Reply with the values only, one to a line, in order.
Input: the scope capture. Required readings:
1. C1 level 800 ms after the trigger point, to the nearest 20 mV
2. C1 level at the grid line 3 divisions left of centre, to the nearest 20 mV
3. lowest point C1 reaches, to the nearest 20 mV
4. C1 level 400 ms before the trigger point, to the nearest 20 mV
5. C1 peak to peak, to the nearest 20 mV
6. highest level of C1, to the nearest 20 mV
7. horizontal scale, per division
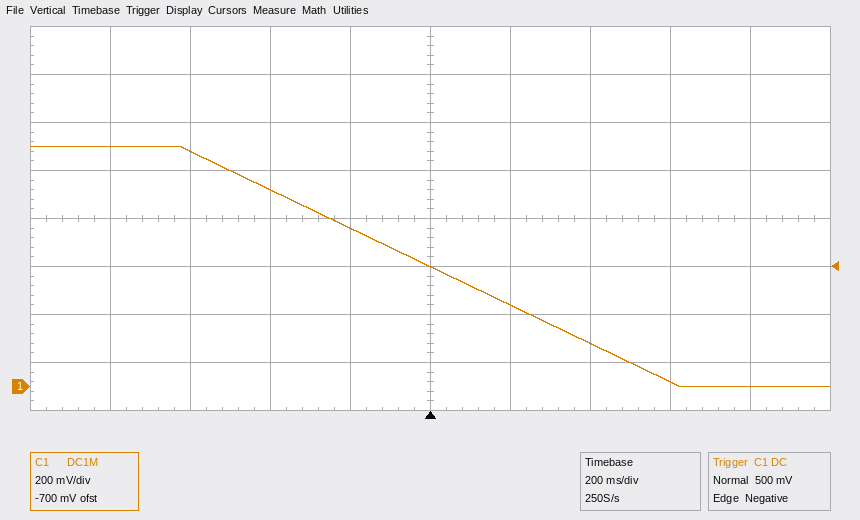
0 mV
980 mV
0 mV
820 mV
1.00 V
1.00 V
200 ms
